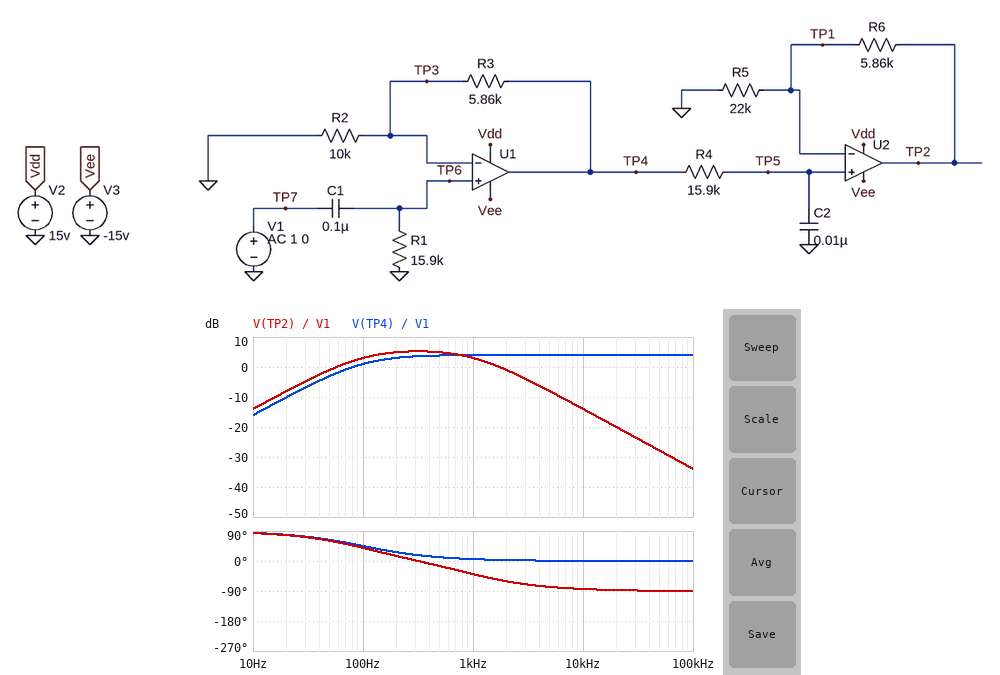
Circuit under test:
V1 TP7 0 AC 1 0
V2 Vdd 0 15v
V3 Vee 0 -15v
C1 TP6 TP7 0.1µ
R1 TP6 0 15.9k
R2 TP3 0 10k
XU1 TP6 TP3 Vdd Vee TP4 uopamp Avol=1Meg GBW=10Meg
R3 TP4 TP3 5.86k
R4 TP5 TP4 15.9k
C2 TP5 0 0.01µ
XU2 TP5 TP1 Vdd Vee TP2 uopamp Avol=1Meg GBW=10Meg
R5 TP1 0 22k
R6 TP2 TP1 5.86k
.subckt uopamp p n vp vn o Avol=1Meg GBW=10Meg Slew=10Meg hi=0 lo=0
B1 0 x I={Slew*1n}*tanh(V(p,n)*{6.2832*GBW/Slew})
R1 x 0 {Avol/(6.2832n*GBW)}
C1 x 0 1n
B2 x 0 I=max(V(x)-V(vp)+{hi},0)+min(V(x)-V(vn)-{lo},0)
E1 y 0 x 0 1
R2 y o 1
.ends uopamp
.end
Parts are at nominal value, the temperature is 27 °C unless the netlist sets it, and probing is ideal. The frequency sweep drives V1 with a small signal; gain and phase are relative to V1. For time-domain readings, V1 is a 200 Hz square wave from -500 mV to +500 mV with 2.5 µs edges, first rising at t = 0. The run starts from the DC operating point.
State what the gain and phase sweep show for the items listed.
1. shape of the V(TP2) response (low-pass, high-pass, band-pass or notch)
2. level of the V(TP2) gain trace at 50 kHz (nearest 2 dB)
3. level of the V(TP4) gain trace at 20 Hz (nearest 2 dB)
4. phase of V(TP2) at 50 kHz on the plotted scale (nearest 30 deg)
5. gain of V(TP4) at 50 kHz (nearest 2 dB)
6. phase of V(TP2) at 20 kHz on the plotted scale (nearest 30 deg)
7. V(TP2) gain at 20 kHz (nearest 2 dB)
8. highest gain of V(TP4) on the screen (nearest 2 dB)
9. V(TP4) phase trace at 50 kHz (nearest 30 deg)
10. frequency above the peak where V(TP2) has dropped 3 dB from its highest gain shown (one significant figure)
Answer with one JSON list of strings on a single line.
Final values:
["band-pass", "-28 dB", "-10 dB", "-90 deg", "4 dB", "-90 deg", "-20 dB", "4 dB", "0 deg", "1 kHz"]
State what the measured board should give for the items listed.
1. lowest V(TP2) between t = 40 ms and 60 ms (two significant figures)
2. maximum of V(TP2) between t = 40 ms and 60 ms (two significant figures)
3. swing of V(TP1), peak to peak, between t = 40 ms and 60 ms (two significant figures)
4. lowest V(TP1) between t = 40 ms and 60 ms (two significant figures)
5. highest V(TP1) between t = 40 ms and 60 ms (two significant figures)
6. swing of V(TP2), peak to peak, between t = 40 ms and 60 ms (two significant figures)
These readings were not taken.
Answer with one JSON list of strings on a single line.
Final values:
["-1.3 V", "1.3 V", "2.0 V", "-1.0 V", "1.0 V", "2.5 V"]
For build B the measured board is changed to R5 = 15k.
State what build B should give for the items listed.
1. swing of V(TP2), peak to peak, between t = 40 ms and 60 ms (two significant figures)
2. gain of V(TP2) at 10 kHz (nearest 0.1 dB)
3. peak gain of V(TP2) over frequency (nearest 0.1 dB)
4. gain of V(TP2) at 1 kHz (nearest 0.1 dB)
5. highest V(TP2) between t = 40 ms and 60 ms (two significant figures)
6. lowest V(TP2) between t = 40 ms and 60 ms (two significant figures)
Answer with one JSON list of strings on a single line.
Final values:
["2.8 V", "-13.2 dB", "6.0 dB", "3.8 dB", "1.4 V", "-1.4 V"]
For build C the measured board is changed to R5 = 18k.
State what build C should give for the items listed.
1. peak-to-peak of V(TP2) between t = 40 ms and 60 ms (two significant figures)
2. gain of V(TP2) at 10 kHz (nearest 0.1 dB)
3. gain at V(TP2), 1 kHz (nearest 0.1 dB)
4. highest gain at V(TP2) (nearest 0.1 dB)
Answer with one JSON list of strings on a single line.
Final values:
["2.6 V", "-13.6 dB", "3.4 dB", "5.6 dB"]
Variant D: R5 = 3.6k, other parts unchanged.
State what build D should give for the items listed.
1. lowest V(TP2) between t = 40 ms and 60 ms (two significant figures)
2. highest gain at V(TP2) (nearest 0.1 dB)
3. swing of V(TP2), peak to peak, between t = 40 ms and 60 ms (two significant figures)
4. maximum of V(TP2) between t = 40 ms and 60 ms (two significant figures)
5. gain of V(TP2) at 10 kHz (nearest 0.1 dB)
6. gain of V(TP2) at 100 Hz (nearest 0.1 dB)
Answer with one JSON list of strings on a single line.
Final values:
["-2.6 V", "11.6 dB", "5.2 V", "2.6 V", "-7.6 dB", "9.3 dB"]
